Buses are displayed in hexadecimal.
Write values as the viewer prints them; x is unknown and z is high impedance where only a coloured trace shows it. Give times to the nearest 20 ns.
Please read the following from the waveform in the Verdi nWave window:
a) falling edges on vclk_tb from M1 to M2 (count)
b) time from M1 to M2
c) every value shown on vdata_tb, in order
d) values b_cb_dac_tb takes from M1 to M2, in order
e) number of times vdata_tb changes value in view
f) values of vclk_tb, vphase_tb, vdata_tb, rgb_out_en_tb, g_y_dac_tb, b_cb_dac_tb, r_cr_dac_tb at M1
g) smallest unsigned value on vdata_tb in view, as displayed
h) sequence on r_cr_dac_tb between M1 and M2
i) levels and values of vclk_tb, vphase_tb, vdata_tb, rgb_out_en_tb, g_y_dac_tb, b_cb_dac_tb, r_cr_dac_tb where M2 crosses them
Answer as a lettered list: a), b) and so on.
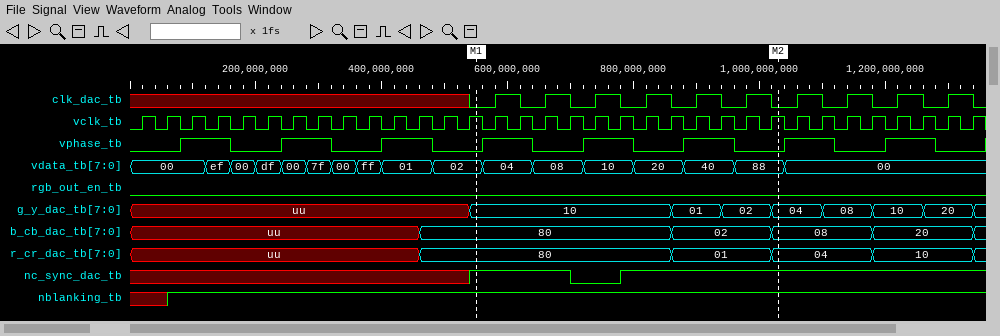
a) 12
b) 480 ns
c) 00, ef, 00, df, 00, 7f, 00, ff, 01, 02, 04, 08, 10, 20, 40, 88, 00
d) 80, 02, 08
e) 16
f) vclk_tb=1, vphase_tb=0, vdata_tb=02, rgb_out_en_tb=0, g_y_dac_tb=10, b_cb_dac_tb=80, r_cr_dac_tb=80
g) 00
h) 80, 01, 04
i) vclk_tb=1, vphase_tb=0, vdata_tb=88, rgb_out_en_tb=0, g_y_dac_tb=04, b_cb_dac_tb=08, r_cr_dac_tb=04
